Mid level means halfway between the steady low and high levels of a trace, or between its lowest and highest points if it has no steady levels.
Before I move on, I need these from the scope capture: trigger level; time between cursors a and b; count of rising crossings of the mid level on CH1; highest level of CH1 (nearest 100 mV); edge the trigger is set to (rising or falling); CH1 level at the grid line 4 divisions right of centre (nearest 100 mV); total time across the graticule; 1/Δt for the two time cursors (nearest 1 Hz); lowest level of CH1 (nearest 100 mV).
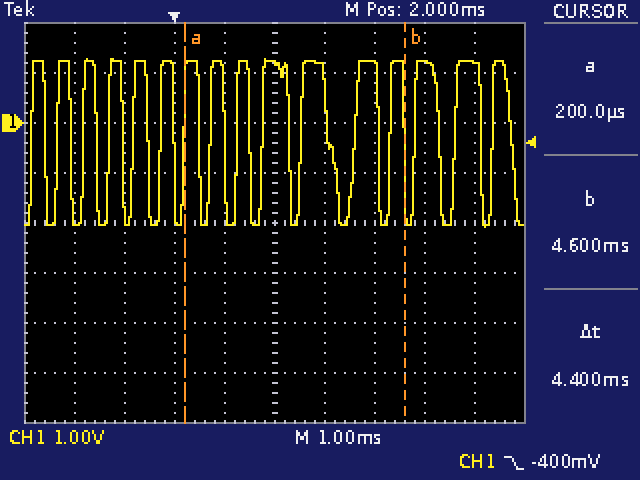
-400 mV
4.4 ms
16
1.3 V
falling
1.2 V
10 ms
227 Hz
-2.1 V
